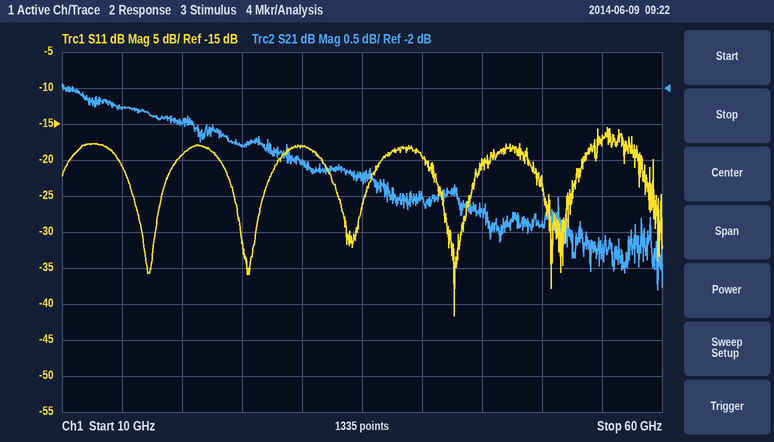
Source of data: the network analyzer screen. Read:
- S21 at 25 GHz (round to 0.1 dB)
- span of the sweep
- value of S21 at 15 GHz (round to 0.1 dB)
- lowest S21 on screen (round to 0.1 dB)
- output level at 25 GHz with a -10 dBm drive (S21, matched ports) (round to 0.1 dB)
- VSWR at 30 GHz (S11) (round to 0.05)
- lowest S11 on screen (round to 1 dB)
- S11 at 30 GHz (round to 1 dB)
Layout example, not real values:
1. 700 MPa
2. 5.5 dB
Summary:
1. -2.8 dB
2. 50 GHz
3. -2.3 dB
4. -4.8 dB
5. -12.8 dBm
6. 1.30
7. -42 dB
8. -18 dB
